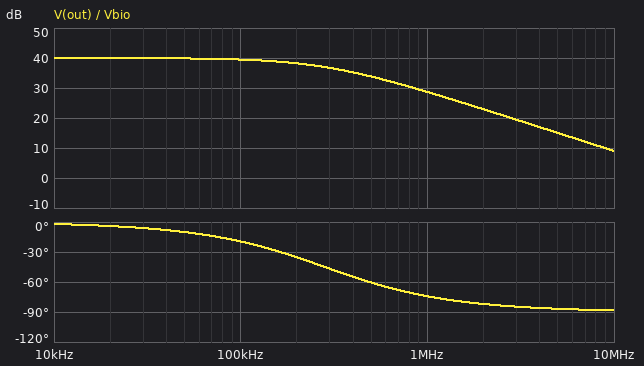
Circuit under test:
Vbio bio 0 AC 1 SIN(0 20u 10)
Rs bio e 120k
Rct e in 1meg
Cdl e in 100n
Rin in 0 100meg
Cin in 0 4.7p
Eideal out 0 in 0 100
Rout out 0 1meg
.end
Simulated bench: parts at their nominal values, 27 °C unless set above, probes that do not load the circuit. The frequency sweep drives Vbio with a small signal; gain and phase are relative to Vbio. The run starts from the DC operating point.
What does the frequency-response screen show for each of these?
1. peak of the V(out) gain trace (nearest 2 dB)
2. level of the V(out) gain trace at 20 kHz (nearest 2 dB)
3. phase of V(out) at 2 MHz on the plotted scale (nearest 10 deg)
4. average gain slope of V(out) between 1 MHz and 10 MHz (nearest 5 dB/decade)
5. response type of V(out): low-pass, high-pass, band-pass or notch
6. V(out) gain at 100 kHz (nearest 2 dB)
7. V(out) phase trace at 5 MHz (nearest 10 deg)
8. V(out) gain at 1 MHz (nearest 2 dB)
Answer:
40 dB
40 dB
-80 deg
-20 dB/decade
low-pass
40 dB
-90 deg
28 dB
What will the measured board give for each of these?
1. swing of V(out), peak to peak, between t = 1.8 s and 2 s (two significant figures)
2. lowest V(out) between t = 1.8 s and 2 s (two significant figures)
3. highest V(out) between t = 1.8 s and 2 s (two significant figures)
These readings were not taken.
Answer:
4.0 mV
-2.0 mV
2.0 mV
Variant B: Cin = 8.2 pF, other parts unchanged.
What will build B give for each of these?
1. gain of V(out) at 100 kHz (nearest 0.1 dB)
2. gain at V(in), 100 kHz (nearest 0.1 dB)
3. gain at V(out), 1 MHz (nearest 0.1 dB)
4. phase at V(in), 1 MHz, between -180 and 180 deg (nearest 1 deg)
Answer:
38.6 dB
-1.4 dB
24.1 dB
-81 deg
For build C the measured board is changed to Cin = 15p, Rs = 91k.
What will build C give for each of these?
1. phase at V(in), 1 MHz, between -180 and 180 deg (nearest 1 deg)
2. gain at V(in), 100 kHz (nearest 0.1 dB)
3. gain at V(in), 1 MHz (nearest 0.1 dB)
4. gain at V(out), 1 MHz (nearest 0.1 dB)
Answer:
-83 deg
-2.4 dB
-18.7 dB
21.3 dB
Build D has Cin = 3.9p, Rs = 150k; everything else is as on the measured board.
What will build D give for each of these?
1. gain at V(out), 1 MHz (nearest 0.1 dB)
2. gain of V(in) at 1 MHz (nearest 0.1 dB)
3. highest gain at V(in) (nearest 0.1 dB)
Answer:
28.4 dB
-11.6 dB
0 dB
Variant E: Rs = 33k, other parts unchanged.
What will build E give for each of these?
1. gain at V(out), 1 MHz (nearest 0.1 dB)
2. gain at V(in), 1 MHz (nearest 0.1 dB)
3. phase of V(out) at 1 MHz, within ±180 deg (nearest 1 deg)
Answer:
37.1 dB
-2.9 dB
-44 deg
